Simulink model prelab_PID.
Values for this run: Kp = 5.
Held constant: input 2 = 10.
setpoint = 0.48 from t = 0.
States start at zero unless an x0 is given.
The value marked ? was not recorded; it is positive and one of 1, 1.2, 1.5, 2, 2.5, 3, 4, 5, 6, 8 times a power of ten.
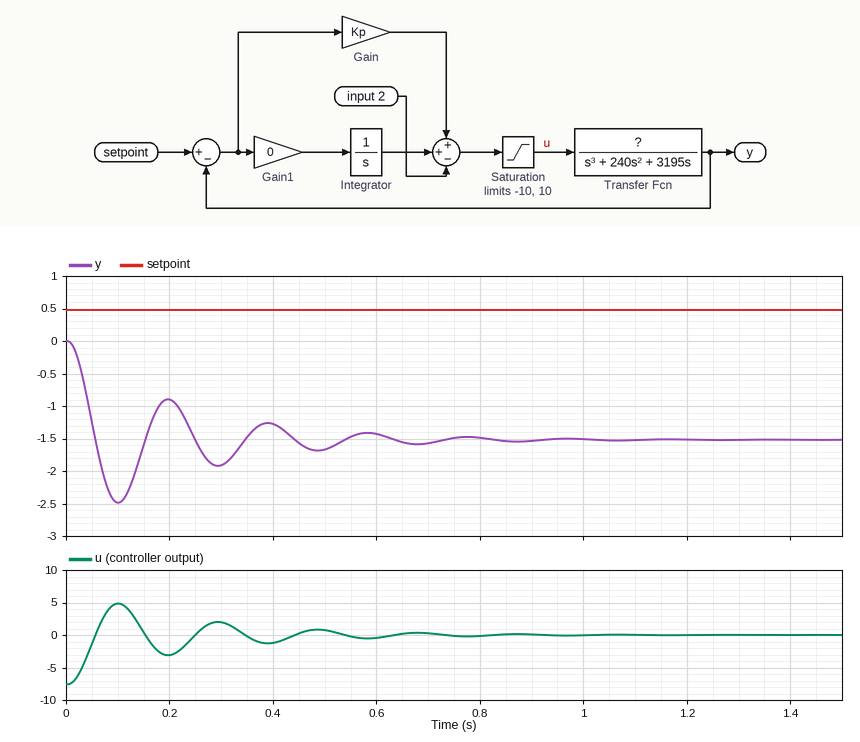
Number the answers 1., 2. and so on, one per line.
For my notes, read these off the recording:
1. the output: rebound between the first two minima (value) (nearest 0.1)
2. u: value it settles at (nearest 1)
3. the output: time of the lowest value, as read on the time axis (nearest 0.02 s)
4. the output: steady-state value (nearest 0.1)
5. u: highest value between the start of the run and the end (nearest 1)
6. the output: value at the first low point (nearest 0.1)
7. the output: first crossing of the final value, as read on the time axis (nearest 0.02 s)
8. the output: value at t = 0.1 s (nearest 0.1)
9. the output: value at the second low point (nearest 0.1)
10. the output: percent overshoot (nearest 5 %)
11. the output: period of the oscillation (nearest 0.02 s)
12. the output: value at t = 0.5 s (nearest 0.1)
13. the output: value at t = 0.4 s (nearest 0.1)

1. -0.9
2. 0
3. 0.10 s
4. -1.5
5. 5
6. -2.5
7. 0.06 s
8. -2.5
9. -1.9
10. 65 %
11. 0.20 s
12. -1.7
13. -1.3
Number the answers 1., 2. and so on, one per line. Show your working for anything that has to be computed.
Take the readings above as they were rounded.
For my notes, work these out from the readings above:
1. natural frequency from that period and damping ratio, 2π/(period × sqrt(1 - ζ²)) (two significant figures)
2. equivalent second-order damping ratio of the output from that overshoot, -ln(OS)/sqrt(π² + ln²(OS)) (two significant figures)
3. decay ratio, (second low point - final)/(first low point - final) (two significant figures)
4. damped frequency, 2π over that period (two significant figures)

1. 2π / (0.2 × sqrt(1 - 0.14²)) = 32 rad/s
2. ln(0.65) = -0.431; 0.431 / sqrt(9.870 + 0.186) = 0.14
3. (-1.9 - (-1.5)) / (-2.5 - (-1.5)) = 0.40
4. 2π / 0.2 = 31 rad/s
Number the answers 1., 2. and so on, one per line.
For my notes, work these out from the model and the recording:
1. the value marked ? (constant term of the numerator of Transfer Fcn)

1. 50000
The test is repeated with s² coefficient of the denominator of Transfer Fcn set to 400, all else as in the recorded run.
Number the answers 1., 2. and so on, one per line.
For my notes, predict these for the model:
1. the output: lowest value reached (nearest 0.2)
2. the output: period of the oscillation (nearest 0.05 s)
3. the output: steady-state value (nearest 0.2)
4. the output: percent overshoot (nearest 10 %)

1. -2.6
2. 0.25 s
3. -1.6
4. 70 %
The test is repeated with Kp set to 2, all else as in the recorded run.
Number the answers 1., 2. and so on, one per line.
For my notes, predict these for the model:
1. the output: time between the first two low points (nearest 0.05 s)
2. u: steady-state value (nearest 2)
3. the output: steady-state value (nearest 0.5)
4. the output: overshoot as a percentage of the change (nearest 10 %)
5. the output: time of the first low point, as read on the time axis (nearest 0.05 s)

1. 0.30 s
2. 0
3. -4.5
4. 40 %
5. 0.15 s
